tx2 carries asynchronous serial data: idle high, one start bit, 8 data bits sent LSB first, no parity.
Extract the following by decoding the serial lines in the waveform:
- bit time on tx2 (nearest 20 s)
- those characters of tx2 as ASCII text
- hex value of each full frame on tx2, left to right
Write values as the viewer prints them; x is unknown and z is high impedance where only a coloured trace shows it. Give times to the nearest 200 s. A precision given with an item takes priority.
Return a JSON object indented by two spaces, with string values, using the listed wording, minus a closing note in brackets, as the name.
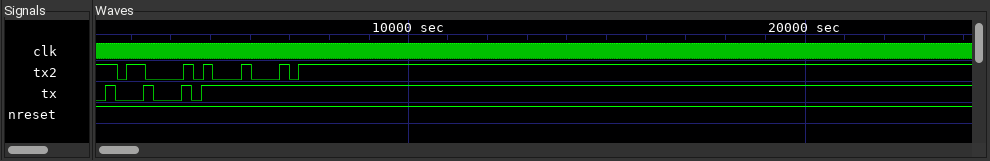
{
  "bit time on tx2": "240 s",
  "those characters of tx2 as ASCII text": "\"CD\"",
  "hex value of each full frame on tx2, left to right": "43, 44"
}
